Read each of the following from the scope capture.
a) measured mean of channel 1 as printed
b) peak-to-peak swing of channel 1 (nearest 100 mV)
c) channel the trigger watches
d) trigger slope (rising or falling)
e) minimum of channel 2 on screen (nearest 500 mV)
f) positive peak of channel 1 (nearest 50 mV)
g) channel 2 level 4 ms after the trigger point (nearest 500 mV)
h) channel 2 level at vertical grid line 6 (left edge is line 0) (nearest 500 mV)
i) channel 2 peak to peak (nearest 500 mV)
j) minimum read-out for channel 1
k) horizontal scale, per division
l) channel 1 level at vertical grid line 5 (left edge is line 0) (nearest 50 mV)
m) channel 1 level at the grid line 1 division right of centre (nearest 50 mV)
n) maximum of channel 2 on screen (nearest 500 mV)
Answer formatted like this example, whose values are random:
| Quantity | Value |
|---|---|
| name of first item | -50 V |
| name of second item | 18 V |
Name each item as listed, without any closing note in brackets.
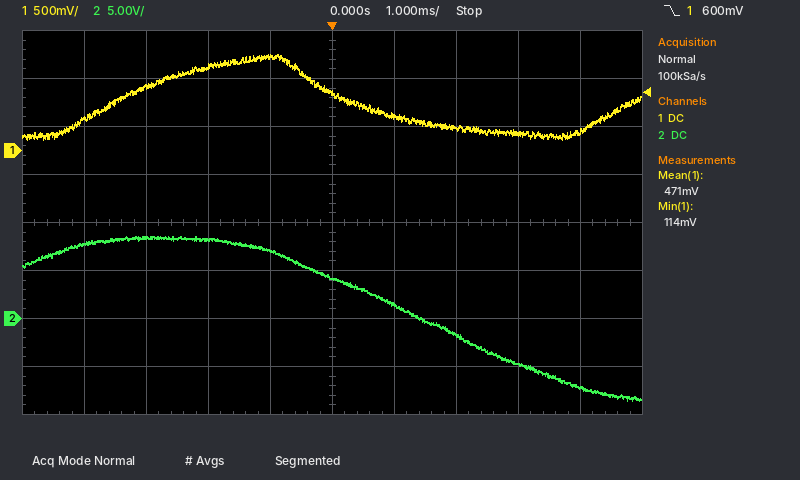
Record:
| Quantity | Value |
|---|---|
| measured mean of channel 1 as printed | 471 mV |
| peak-to-peak swing of channel 1 | 900 mV |
| channel the trigger watches | channel 1 |
| trigger slope | falling |
| minimum of channel 2 on screen | -8.5 V |
| positive peak of channel 1 | 1.00 V |
| channel 2 level 4 ms after the trigger point | -7.0 V |
| channel 2 level at vertical grid line 6 (left edge is line 0) | 1.5 V |
| channel 2 peak to peak | 17.0 V |
| minimum read-out for channel 1 | 114 mV |
| horizontal scale, per division | 1 ms |
| channel 1 level at vertical grid line 5 (left edge is line 0) | 600 mV |
| channel 1 level at the grid line 1 division right of centre | 350 mV |
| maximum of channel 2 on screen | 8.5 V |
